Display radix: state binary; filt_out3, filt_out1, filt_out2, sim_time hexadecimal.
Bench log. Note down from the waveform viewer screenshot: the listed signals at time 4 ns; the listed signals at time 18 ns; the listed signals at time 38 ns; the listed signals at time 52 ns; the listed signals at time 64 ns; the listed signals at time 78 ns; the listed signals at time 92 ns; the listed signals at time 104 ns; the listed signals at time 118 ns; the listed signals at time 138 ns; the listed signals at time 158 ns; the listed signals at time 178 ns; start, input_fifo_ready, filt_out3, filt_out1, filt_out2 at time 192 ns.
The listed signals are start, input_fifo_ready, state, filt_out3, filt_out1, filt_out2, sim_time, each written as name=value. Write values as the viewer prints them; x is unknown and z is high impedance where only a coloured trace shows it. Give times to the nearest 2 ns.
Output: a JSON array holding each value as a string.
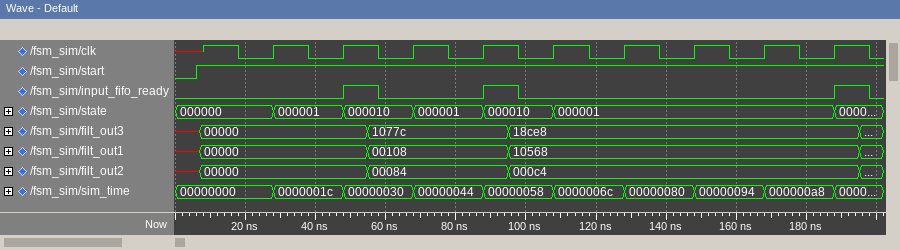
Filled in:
["start=0, input_fifo_ready=0, state=000000, filt_out3=x, filt_out1=x, filt_out2=x, sim_time=00000000", "start=1, input_fifo_ready=0, state=000000, filt_out3=00000, filt_out1=00000, filt_out2=00000, sim_time=00000000", "start=1, input_fifo_ready=0, state=000001, filt_out3=00000, filt_out1=00000, filt_out2=00000, sim_time=0000001c", "start=1, input_fifo_ready=1, state=000010, filt_out3=00000, filt_out1=00000, filt_out2=00000, sim_time=00000030", "start=1, input_fifo_ready=0, state=000010, filt_out3=1077c, filt_out1=00108, filt_out2=00084, sim_time=00000030", "start=1, input_fifo_ready=0, state=000001, filt_out3=1077c, filt_out1=00108, filt_out2=00084, sim_time=00000044", "start=1, input_fifo_ready=1, state=000010, filt_out3=1077c, filt_out1=00108, filt_out2=00084, sim_time=00000058", "start=1, input_fifo_ready=0, state=000010, filt_out3=18ce8, filt_out1=10568, filt_out2=000c4, sim_time=00000058", "start=1, input_fifo_ready=0, state=000001, filt_out3=18ce8, filt_out1=10568, filt_out2=000c4, sim_time=0000006c", "start=1, input_fifo_ready=0, state=000001, filt_out3=18ce8, filt_out1=10568, filt_out2=000c4, sim_time=00000080", "start=1, input_fifo_ready=0, state=000001, filt_out3=18ce8, filt_out1=10568, filt_out2=000c4, sim_time=00000094", "start=1, input_fifo_ready=0, state=000001, filt_out3=18ce8, filt_out1=10568, filt_out2=000c4, sim_time=000000a8", "start=1, input_fifo_ready=1, filt_out3=18ce8, filt_out1=10568, filt_out2=000c4"]
